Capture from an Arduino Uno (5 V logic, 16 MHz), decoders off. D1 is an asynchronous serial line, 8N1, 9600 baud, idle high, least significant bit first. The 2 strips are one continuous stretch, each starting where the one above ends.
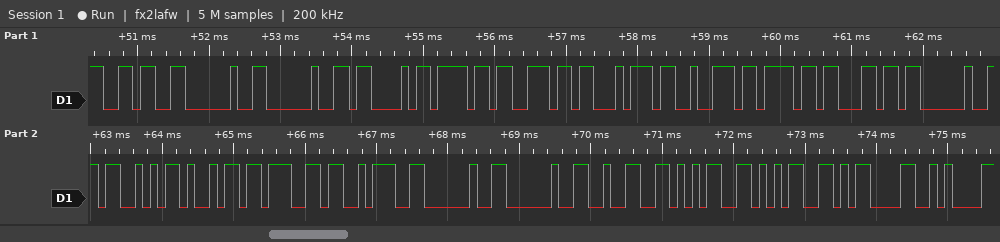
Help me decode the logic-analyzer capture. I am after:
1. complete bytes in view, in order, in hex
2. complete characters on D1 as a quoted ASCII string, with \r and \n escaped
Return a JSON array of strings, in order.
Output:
["36 20 20 43 6F 6E 74 72 6F 6C 20 53 69 67 3A 20 20 32 35 35 0D 0A", "\"6  Control Sig:  255\\r\\n\""]
